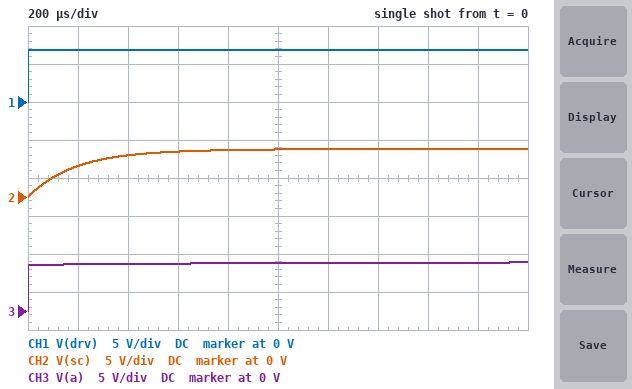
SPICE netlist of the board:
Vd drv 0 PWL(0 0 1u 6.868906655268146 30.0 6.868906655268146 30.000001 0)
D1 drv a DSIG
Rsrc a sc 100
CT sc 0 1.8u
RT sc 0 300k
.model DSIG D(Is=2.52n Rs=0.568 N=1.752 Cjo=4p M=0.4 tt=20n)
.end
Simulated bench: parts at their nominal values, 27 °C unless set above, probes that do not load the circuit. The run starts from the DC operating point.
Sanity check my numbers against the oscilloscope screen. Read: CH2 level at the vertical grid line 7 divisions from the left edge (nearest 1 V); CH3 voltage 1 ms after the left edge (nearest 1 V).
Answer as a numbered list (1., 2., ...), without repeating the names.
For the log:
1. 6 V
2. 6 V
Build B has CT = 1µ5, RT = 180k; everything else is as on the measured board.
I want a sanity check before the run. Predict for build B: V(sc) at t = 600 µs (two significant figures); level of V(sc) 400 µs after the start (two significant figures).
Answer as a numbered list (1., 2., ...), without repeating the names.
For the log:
1. 6.1 V
2. 5.7 V
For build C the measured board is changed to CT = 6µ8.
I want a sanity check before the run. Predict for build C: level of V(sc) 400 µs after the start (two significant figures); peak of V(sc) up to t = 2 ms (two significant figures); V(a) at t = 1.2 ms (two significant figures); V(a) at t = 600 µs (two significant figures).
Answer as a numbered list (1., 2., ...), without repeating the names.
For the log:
1. 2.7 V
2. 5.9 V
3. 6.2 V
4. 6.1 V
